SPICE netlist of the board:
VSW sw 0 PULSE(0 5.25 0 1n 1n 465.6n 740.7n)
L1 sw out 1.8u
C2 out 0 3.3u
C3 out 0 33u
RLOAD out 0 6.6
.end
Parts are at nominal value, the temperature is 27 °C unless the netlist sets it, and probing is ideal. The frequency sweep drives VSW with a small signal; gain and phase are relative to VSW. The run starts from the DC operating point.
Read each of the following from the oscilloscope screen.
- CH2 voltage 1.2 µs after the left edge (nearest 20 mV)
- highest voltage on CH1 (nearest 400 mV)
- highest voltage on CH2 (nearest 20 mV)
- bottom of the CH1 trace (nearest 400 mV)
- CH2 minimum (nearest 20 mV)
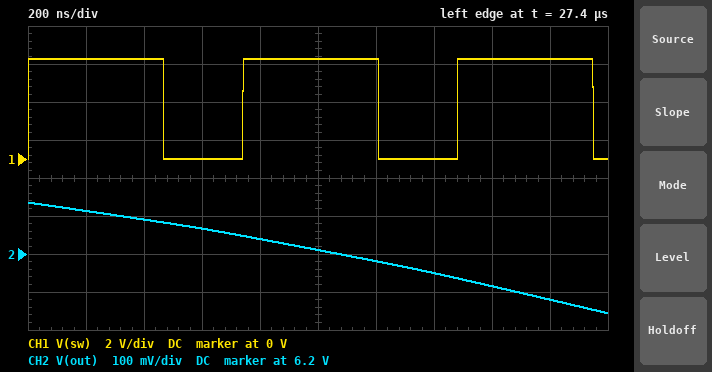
6.18 V
5.2 V
6.34 V
0 V
6.04 V
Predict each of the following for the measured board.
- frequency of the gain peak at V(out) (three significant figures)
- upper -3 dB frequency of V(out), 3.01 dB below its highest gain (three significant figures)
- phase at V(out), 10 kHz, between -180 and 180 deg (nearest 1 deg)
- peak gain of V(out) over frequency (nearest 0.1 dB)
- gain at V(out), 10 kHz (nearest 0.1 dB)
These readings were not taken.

19.7 kHz
20.0 kHz
-1 deg
29.4 dB
2.6 dB
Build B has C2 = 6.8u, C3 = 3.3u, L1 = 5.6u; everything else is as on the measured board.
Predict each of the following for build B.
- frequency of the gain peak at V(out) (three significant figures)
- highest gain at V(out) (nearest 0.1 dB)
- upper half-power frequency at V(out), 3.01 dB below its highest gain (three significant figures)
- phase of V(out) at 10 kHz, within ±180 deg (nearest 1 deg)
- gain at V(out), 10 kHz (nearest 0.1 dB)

21.1 kHz
19.0 dB
22.3 kHz
-4 deg
2.2 dB
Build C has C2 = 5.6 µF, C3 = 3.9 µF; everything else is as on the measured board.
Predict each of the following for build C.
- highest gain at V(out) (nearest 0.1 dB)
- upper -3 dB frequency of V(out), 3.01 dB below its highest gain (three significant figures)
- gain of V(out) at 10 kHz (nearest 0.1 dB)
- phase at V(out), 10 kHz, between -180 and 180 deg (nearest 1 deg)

23.6 dB
39.7 kHz
0.6 dB
-1 deg
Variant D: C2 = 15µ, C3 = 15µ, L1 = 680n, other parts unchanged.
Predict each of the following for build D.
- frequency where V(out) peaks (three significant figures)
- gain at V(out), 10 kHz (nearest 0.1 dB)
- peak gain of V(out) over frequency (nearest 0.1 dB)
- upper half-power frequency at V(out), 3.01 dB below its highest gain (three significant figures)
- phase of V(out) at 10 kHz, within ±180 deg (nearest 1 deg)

35.2 kHz
0.7 dB
32.8 dB
35.6 kHz
0 deg
